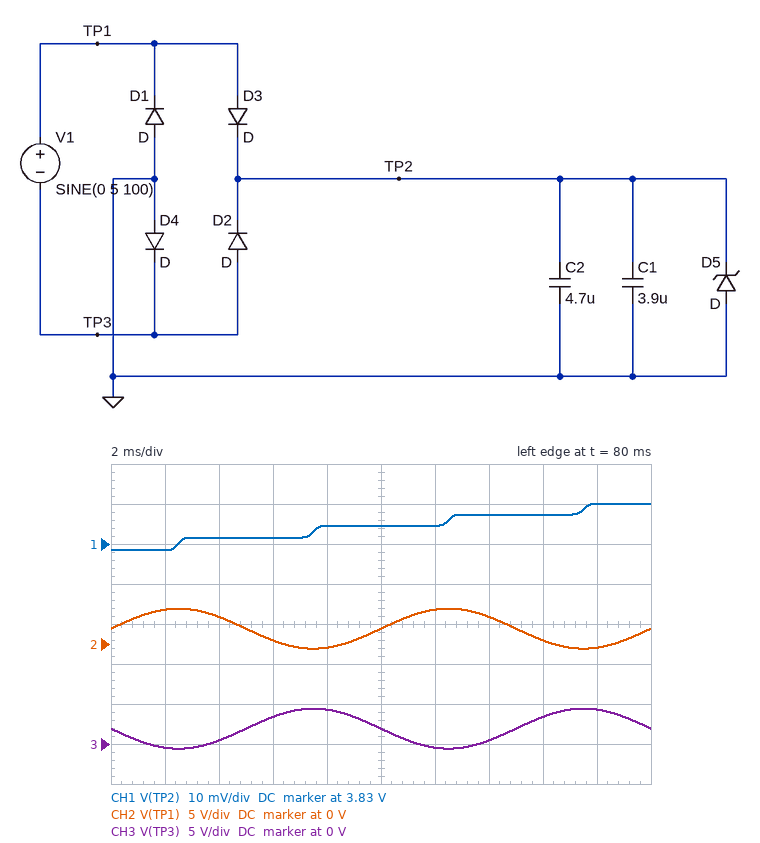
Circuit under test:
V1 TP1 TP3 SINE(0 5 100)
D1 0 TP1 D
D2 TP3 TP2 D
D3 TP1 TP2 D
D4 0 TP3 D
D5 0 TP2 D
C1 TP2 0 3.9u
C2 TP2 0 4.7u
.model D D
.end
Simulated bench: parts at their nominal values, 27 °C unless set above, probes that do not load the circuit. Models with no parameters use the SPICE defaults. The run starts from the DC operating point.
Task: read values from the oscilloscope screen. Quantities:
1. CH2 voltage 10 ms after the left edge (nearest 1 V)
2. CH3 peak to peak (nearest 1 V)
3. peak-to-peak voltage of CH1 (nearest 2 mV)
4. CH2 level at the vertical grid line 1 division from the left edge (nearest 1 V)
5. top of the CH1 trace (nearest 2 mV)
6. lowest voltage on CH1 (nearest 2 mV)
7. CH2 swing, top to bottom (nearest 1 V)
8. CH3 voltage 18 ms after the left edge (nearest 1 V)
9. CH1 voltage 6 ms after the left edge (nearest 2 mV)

2 V
5 V
12 mV
4 V
3.840 V
3.828 V
5 V
4 V
3.832 V
